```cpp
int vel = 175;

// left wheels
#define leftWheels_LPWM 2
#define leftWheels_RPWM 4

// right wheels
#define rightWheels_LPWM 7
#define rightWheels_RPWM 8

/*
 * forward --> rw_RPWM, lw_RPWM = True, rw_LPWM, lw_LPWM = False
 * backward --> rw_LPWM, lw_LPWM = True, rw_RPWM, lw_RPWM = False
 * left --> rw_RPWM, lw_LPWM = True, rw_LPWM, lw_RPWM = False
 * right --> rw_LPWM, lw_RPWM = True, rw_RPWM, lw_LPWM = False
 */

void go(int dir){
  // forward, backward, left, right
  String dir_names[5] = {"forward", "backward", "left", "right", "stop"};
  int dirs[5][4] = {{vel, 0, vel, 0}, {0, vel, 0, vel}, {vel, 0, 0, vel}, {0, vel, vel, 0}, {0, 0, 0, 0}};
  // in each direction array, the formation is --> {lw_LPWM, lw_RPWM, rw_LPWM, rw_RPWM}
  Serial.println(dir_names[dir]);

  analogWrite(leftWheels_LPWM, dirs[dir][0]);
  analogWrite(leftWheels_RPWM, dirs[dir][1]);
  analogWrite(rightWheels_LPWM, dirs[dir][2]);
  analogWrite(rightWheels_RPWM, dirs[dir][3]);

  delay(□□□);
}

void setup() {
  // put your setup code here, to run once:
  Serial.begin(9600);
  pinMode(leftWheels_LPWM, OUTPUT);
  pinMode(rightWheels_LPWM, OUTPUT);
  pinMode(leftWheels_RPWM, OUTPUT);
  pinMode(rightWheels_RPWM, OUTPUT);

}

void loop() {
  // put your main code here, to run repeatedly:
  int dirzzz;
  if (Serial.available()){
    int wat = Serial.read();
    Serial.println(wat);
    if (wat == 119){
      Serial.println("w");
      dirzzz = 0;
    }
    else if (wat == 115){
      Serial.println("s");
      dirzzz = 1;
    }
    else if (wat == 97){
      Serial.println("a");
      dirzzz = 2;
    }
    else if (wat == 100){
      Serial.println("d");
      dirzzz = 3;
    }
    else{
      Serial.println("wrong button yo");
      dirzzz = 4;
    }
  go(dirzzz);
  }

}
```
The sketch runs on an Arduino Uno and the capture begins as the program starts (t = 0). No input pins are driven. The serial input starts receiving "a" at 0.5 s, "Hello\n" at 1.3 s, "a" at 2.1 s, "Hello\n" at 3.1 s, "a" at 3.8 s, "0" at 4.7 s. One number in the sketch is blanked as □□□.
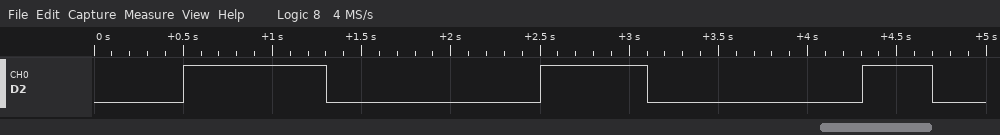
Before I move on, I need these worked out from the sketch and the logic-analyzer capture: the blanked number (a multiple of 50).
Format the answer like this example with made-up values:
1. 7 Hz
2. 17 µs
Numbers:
1. 200
